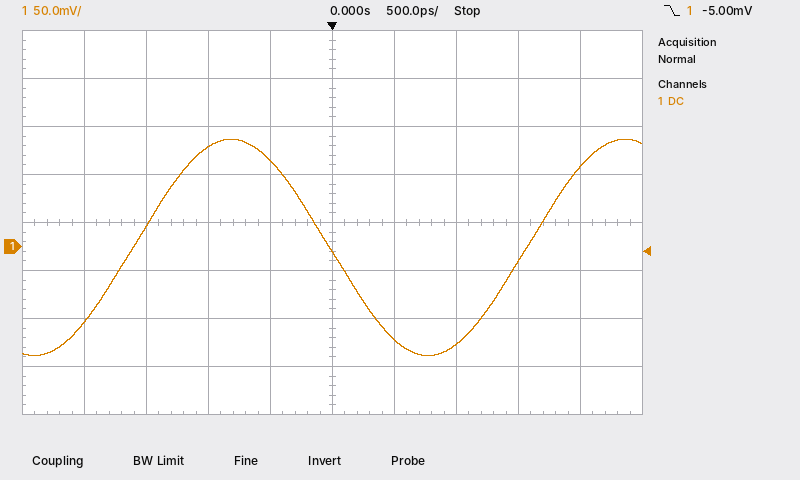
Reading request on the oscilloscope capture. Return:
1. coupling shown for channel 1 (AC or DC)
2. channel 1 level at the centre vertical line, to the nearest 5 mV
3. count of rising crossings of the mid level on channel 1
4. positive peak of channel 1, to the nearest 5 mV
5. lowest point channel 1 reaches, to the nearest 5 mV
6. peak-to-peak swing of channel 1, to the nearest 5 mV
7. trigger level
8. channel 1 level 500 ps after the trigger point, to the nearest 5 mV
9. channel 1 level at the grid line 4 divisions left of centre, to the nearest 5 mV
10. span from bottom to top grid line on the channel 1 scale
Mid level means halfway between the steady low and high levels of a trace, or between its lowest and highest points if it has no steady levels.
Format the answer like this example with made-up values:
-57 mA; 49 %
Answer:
DC; -5 mV; 2; 110 mV; -115 mV; 225 mV; -5.00 mV; -95 mV; -80 mV; 400 mV
